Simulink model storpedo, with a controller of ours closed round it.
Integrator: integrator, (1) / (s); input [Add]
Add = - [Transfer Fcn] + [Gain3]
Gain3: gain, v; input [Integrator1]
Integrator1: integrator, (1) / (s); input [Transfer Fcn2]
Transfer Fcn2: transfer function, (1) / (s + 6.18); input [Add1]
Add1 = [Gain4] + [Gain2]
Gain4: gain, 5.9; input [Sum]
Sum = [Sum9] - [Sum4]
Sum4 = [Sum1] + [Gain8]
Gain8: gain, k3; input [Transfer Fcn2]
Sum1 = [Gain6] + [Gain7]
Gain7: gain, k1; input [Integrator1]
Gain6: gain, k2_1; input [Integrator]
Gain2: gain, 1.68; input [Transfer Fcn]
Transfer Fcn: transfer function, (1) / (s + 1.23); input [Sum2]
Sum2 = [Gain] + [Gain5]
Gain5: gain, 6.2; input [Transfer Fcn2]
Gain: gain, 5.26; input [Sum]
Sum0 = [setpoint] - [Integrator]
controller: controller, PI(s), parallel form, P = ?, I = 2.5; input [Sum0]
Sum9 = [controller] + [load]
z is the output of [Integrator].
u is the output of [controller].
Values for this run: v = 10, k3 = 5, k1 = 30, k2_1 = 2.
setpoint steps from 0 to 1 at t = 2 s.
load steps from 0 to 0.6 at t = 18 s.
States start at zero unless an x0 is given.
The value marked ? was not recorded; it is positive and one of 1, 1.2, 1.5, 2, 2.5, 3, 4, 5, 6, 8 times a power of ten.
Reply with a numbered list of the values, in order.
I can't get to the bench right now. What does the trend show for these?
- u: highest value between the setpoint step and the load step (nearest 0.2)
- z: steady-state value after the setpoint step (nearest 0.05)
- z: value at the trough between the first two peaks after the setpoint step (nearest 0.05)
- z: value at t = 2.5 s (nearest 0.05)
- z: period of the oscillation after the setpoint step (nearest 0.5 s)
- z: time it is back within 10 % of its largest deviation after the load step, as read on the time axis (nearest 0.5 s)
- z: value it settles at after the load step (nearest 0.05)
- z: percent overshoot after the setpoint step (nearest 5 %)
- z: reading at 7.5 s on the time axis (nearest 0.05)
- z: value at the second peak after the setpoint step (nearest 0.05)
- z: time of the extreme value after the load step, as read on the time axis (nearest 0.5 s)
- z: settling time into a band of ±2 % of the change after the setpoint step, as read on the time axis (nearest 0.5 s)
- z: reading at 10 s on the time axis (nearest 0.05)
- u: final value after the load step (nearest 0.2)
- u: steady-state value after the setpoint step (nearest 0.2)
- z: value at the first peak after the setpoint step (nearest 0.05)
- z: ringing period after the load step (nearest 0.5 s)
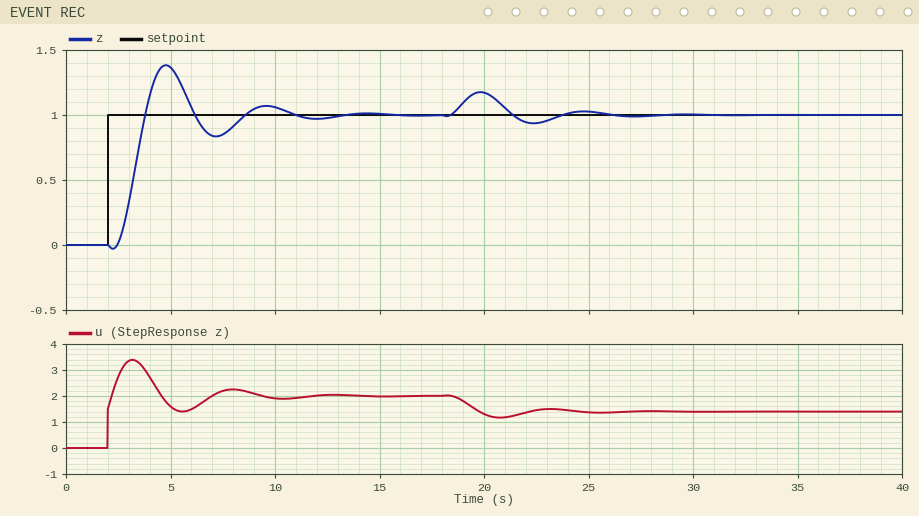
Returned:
1. 3.4
2. 1.00
3. 0.85
4. 0.00
5. 5.0 s
6. 25.5 s
7. 1.00
8. 40 %
9. 0.85
10. 1.05
11. 20.0 s
12. 12.5 s
13. 1.05
14. 1.4
15. 2.0
16. 1.40
17. 5.0 s
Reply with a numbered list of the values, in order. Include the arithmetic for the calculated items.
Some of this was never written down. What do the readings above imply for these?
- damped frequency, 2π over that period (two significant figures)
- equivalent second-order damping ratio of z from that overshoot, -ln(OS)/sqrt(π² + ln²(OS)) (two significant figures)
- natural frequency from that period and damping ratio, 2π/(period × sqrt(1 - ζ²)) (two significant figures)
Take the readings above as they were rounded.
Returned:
1. 2π / 5 = 1.3 rad/s
2. ln(0.4) = -0.916; 0.916 / sqrt(9.870 + 0.840) = 0.28
3. 2π / (5 × sqrt(1 - 0.28²)) = 1.3 rad/s
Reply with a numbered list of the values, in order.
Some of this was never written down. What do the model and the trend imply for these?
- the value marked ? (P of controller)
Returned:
1. 1.5
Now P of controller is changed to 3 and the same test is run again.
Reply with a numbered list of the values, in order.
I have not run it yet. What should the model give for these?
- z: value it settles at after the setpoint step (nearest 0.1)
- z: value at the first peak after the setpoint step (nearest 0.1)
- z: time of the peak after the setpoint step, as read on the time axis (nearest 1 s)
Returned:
1. 1.0
2. 1.3
3. 4 s
